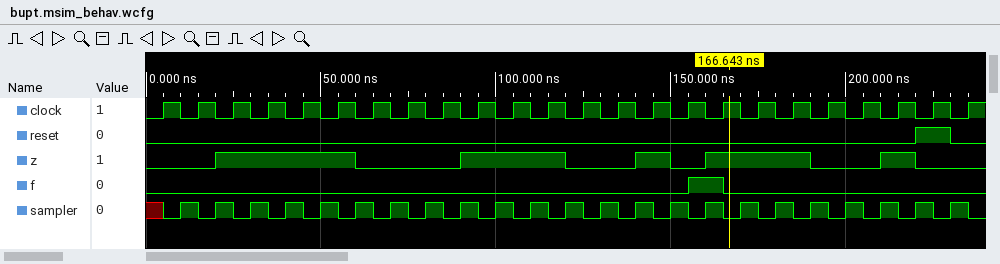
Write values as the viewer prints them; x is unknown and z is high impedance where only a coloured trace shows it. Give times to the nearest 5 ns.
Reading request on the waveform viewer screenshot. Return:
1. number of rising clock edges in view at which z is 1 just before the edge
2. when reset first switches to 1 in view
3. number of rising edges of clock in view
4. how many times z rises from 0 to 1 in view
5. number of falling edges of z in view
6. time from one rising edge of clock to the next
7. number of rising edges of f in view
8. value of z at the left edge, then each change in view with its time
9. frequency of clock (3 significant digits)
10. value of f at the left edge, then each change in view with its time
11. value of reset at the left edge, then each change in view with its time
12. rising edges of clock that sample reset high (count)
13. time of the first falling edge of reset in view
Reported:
12
220 ns
24
5
5
10 ns
1
0, 1 at 20 ns, 0 at 60 ns, 1 at 90 ns, 0 at 120 ns, 1 at 140 ns, 0 at 150 ns, 1 at 160 ns, 0 at 190 ns, 1 at 210 ns, 0 at 220 ns
100 MHz
0, 1 at 155 ns, 0 at 165 ns
0, 1 at 220 ns, 0 at 230 ns
1
230 ns
